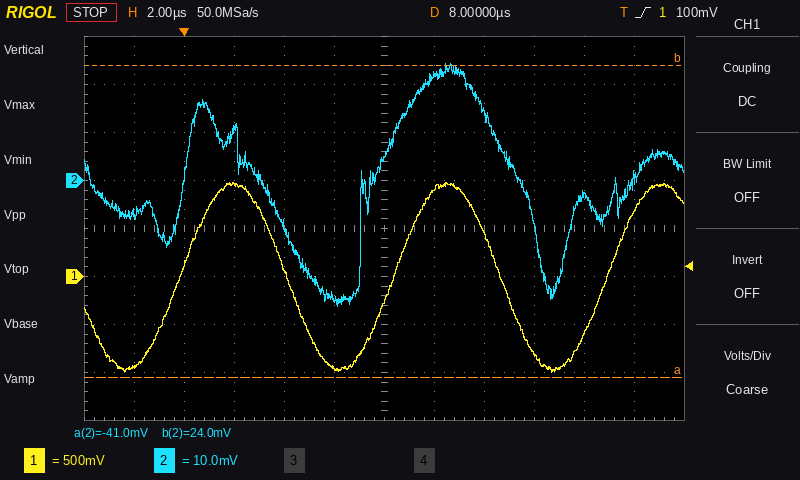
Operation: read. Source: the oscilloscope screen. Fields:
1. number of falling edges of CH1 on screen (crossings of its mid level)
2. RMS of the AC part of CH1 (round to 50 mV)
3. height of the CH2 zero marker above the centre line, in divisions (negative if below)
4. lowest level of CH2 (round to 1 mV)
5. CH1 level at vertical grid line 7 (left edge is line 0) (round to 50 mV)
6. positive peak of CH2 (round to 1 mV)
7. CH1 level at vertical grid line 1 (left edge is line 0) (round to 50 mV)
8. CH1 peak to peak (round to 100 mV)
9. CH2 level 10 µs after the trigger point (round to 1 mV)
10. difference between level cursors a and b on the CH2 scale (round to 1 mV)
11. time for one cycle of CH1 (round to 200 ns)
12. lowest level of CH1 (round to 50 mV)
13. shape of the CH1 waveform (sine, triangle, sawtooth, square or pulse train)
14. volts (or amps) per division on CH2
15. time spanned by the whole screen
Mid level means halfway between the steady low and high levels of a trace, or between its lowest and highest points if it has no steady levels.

2
700 mV
+1.0 div
-26 mV
900 mV
24 mV
-950 mV
2.00 V
22 mV
65 mV
8.6 µs
-1.00 V
sine
10 mV
24 µs
